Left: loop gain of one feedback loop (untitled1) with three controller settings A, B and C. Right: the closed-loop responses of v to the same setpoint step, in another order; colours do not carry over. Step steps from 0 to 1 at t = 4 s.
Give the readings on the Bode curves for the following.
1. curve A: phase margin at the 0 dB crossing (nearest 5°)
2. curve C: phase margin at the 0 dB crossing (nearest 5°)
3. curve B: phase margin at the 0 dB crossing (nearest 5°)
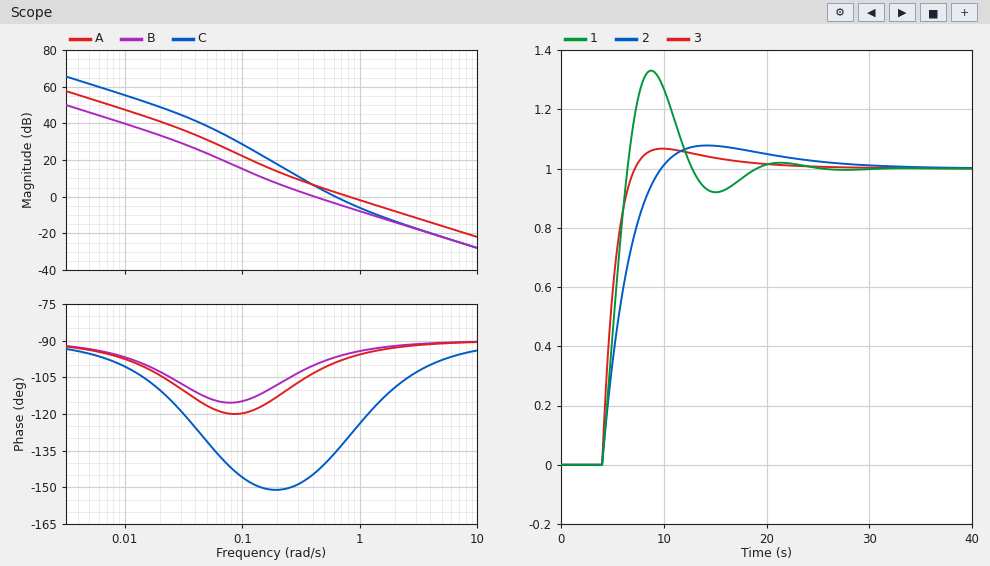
85°
45°
80°
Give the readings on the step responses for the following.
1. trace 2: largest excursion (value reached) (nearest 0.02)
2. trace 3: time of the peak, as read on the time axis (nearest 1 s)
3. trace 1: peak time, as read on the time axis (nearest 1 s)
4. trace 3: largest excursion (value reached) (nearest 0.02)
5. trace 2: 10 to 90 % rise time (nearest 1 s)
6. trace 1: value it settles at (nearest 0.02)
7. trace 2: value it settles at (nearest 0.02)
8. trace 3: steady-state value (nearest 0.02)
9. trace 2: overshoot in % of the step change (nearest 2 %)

1.08
10 s
9 s
1.06
4 s
1.00
1.00
1.00
8 %
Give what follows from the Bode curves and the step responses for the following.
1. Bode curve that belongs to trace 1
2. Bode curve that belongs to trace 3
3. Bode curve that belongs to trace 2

C
A
B
